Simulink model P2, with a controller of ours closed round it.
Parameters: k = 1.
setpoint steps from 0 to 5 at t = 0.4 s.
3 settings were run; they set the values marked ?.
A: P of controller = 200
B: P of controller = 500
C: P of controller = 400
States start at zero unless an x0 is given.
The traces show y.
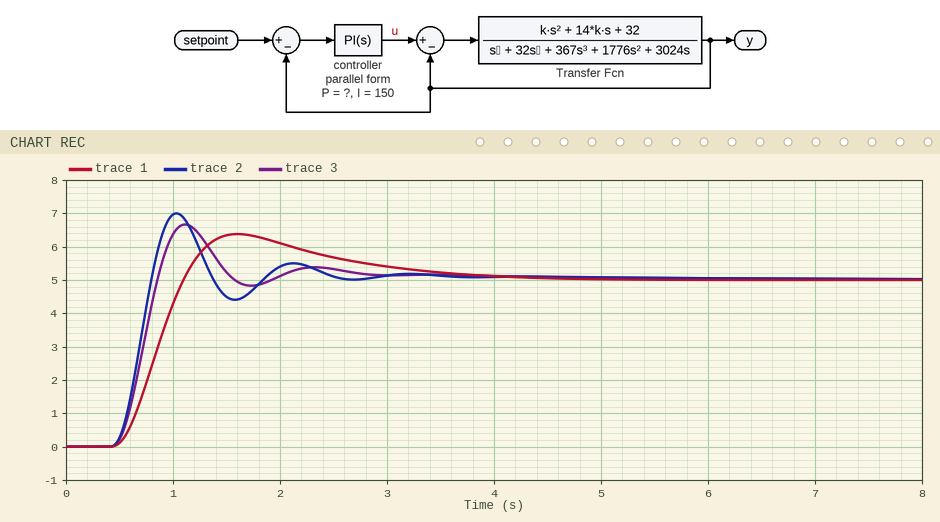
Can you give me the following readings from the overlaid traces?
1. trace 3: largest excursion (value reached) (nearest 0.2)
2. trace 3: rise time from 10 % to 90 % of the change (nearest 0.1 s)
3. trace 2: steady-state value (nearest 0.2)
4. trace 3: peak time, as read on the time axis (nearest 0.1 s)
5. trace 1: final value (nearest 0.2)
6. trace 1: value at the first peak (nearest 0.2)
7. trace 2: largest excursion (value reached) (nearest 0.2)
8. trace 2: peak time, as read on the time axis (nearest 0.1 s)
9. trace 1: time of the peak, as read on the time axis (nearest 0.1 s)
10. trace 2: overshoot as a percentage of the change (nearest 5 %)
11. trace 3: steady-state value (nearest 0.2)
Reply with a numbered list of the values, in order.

1. 6.6
2. 0.3 s
3. 5.0
4. 1.1 s
5. 5.0
6. 6.4
7. 7.0
8. 1.0 s
9. 1.6 s
10. 40 %
11. 5.0
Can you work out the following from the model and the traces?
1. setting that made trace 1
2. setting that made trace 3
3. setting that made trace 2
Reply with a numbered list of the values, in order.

1. A
2. C
3. B
